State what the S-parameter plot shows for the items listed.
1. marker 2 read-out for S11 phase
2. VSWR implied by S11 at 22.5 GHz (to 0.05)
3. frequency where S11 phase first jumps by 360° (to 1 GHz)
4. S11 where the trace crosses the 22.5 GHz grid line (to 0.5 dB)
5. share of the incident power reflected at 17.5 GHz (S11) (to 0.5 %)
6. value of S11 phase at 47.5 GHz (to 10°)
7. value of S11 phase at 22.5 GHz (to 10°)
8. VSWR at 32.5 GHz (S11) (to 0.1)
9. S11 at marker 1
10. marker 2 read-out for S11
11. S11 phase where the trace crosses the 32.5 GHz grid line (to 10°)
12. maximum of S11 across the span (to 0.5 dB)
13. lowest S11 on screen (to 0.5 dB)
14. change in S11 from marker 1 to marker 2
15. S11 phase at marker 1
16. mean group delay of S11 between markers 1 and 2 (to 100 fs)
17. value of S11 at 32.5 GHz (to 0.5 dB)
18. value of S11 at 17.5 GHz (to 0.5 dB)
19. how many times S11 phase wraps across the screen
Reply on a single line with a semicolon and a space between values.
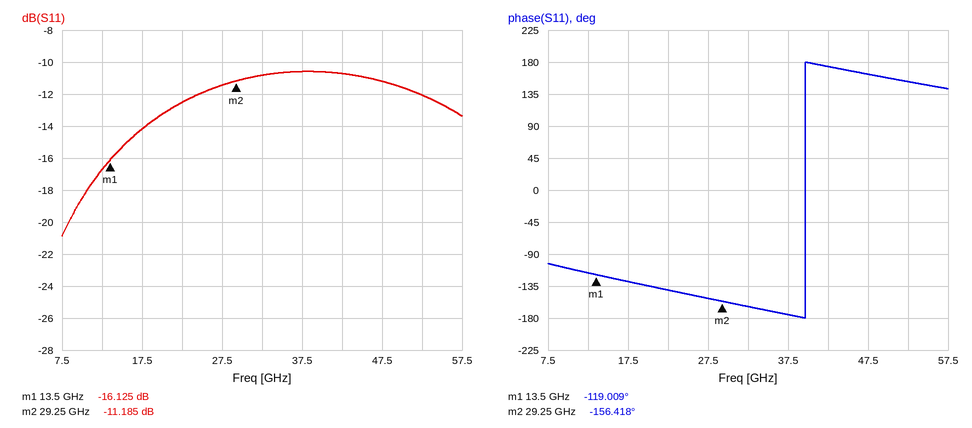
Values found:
-156.418°; 1.60; 40 GHz; -12.5 dB; 4.0 %; 160°; -140°; 1.8; -16.125 dB; -11.185 dB; -160°; -10.5 dB; -21.0 dB; 4.940 dB; -119.009°; 6.6 ps; -11.0 dB; -14.0 dB; 1
